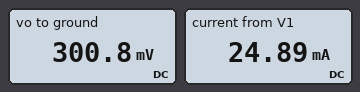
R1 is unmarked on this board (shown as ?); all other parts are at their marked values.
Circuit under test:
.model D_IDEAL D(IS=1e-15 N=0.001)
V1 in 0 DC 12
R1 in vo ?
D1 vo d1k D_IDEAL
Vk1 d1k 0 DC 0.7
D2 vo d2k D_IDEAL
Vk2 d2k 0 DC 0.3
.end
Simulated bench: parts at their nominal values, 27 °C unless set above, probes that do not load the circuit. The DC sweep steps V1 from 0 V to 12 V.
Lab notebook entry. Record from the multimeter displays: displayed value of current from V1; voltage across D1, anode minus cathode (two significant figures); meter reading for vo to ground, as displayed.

24.89 mA
-400 mV
300.8 mV
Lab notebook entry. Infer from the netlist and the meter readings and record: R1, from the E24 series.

470 Ω
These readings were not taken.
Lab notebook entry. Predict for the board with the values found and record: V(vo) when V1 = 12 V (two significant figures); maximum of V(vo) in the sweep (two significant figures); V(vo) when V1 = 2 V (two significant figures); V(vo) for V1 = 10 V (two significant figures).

300 mV
300 mV
300 mV
300 mV
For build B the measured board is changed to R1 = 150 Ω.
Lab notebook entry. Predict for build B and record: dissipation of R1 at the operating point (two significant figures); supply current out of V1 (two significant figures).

910 mW
78 mA
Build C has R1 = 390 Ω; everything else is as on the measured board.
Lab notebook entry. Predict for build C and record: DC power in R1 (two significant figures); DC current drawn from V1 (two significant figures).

350 mW
30 mA
